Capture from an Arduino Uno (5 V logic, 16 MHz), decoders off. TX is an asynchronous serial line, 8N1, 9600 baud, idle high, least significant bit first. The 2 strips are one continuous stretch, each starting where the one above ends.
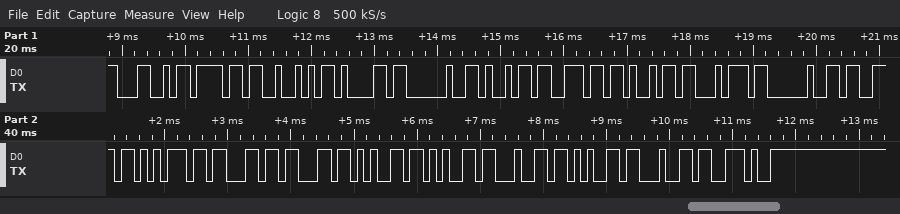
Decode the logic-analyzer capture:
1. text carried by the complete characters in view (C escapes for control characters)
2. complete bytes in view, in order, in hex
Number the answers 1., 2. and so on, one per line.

1. "LoRa init succeeded."
2. 0x4C 0x6F 0x52 0x61 0x20 0x69 0x6E 0x69 0x74 0x20 0x73 0x75 0x63 0x63 0x65 0x65 0x64 0x65 0x64 0x2E
